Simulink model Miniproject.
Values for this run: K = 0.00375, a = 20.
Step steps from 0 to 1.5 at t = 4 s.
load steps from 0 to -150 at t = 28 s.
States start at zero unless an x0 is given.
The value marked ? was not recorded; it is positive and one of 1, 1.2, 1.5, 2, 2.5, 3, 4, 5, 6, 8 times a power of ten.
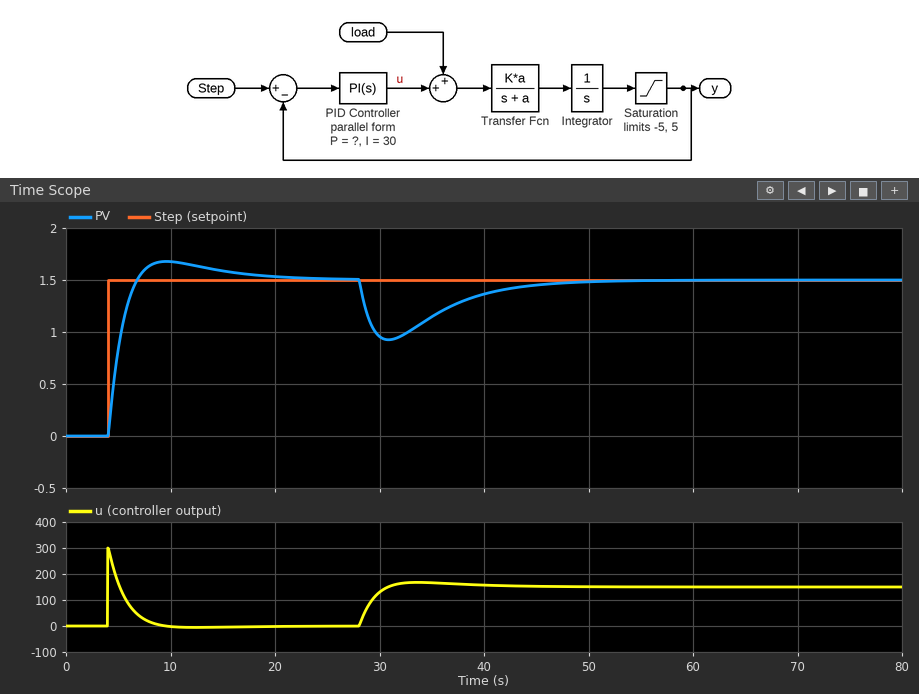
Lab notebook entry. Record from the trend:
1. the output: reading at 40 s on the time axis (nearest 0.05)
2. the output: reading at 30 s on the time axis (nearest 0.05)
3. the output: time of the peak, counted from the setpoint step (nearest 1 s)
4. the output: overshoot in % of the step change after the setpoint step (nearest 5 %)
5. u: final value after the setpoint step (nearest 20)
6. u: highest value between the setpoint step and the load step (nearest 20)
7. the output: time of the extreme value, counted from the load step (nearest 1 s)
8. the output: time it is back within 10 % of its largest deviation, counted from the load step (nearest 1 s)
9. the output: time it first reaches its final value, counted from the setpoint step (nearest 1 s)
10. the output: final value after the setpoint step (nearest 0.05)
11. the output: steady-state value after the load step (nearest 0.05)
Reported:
1.35
0.95
6 s
10 %
0
300
3 s
16 s
3 s
1.50
1.50
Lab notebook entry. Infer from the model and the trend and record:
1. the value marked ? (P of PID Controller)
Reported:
200
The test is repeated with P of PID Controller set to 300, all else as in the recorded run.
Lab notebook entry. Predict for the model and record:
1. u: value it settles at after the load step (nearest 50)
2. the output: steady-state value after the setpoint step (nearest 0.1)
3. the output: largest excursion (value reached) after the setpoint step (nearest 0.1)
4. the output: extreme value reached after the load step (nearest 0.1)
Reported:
150
1.5
1.6
1.1
